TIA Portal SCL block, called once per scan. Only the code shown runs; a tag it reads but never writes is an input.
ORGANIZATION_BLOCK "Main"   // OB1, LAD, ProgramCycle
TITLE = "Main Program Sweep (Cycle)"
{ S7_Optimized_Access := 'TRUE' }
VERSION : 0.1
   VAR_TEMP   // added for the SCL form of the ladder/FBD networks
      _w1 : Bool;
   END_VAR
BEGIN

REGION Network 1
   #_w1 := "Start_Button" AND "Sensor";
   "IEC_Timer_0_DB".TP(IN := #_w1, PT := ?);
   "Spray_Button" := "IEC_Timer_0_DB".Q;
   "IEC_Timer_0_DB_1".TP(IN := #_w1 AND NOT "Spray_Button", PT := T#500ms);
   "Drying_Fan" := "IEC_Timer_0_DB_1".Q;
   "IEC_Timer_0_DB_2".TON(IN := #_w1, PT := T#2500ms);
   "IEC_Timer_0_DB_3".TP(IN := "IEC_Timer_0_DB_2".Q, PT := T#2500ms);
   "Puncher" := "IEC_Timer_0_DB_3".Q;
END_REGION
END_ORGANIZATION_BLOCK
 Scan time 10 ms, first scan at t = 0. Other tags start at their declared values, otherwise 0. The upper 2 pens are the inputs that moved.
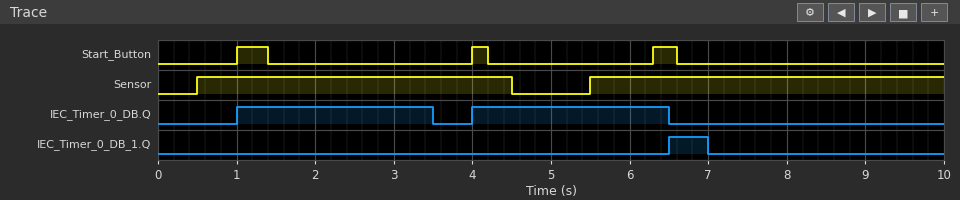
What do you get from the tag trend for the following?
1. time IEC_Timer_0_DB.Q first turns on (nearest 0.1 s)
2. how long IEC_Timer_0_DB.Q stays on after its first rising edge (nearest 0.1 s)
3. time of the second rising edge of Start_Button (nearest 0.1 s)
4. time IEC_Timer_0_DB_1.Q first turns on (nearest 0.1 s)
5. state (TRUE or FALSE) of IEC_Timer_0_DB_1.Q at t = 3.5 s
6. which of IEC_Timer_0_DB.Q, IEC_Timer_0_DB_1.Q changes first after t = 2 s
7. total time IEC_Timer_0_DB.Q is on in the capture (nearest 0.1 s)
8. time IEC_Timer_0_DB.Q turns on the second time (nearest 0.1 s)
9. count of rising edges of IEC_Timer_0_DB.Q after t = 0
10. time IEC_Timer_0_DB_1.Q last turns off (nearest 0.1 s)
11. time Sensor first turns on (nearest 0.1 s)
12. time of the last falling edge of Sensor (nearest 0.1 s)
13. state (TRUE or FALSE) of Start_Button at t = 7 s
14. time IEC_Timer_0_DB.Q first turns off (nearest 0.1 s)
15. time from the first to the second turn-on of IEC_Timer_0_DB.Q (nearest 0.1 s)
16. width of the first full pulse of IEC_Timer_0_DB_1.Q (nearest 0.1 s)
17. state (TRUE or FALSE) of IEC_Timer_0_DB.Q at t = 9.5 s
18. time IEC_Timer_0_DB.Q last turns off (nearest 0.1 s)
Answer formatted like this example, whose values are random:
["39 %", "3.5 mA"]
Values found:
["1.0 s", "2.5 s", "4.0 s", "6.5 s", "FALSE", "IEC_Timer_0_DB.Q", "5.0 s", "4.0 s", "2", "7.0 s", "0.5 s", "4.5 s", "FALSE", "3.5 s", "3.0 s", "0.5 s", "FALSE", "6.5 s"]
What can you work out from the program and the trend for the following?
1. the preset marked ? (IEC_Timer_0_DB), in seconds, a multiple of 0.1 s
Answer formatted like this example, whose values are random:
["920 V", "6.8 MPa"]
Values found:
["2.5 s"]
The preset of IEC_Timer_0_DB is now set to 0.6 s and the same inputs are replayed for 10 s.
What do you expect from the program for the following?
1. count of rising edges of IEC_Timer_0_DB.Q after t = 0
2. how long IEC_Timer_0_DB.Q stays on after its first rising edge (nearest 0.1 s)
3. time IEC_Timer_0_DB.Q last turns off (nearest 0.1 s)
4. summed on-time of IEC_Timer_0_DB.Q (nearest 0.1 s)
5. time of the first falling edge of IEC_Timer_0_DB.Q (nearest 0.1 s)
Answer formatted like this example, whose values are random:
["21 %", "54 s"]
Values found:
["3", "0.6 s", "6.9 s", "1.8 s", "1.6 s"]
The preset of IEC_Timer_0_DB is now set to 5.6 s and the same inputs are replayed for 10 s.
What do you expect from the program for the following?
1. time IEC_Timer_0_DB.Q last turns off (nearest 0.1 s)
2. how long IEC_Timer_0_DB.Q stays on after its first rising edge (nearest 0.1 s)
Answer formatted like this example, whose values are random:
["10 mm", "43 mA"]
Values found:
["6.6 s", "5.6 s"]
